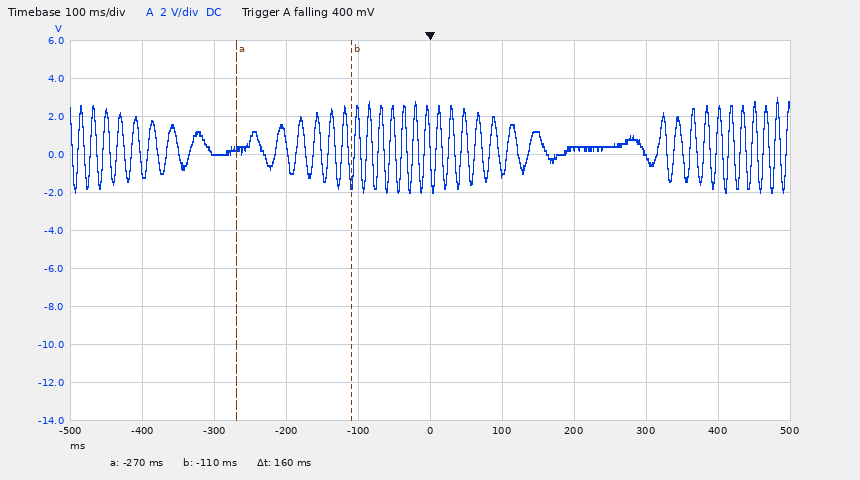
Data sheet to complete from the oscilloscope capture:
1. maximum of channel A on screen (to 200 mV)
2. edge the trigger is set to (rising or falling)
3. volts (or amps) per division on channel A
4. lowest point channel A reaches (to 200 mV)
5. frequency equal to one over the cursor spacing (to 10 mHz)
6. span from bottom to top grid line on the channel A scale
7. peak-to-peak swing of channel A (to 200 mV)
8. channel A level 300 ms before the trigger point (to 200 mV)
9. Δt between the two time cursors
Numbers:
3.0 V
falling
2 V
-2.0 V
6.25 Hz
20 V
5.0 V
0.0 V
160 ms
